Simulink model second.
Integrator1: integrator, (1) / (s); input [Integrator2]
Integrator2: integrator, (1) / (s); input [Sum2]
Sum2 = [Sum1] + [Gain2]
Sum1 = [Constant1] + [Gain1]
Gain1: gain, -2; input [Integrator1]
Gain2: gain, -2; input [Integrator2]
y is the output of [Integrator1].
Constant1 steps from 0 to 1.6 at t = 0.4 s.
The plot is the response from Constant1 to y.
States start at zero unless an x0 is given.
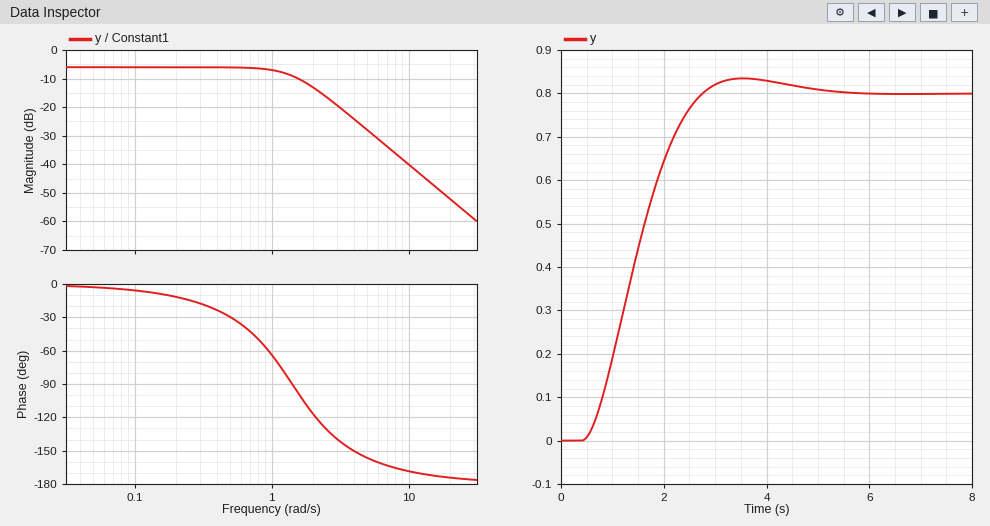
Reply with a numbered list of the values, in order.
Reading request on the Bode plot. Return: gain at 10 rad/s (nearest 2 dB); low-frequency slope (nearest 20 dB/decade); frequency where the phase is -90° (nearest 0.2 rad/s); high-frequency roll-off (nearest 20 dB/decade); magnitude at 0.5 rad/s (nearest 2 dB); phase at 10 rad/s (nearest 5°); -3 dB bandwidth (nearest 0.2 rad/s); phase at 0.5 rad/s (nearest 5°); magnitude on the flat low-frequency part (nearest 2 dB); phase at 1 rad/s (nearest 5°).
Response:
1. -40 dB
2. 0 dB/decade
3. 1.4 rad/s
4. -40 dB/decade
5. -6 dB
6. -170°
7. 1.4 rad/s
8. -30°
9. -6 dB
10. -65°
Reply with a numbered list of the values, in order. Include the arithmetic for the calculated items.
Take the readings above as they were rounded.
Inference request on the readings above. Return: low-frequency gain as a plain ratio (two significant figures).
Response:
1. 10^(-6 / 20) = 0.50
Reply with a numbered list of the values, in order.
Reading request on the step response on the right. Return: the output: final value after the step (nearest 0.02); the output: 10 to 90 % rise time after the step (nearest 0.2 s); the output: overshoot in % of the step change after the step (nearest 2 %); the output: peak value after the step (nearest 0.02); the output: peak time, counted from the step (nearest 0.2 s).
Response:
1. 0.80
2. 1.6 s
3. 4 %
4. 0.84
5. 3.2 s
